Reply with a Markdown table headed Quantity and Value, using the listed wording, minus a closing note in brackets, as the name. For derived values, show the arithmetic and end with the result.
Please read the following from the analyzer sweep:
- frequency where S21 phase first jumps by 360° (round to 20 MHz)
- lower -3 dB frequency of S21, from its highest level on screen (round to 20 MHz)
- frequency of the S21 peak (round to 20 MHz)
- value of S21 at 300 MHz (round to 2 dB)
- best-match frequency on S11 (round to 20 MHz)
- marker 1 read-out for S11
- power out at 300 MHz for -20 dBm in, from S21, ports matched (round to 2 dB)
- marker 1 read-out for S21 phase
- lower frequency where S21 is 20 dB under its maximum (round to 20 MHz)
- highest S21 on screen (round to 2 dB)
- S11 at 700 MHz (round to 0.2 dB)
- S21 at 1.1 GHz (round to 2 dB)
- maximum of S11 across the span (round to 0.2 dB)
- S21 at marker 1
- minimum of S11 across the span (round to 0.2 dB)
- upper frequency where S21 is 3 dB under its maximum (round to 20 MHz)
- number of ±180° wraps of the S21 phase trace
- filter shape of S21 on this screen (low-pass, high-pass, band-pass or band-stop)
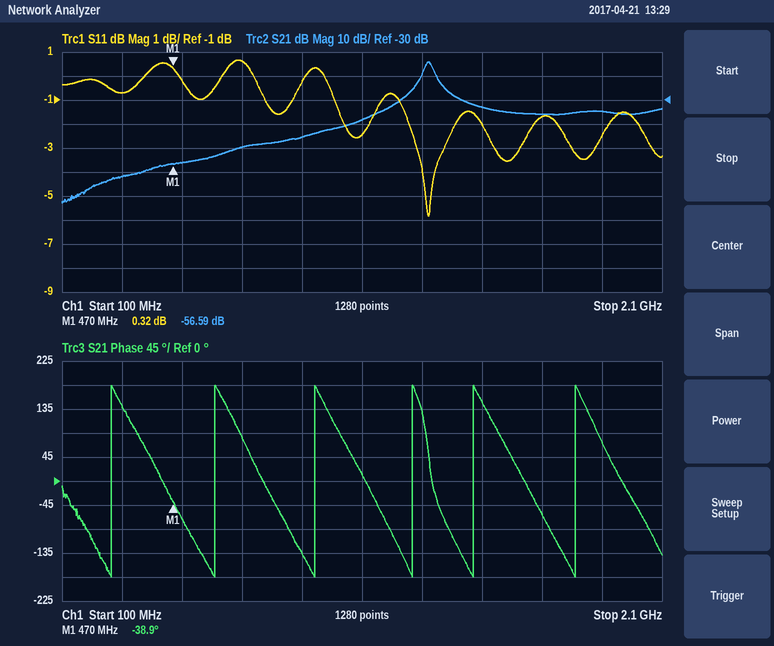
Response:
| Quantity | Value |
|---|---|
| frequency where S21 phase first jumps by 360° | 260 MHz |
| lower -3 dB frequency of S21, from its highest level on screen | 1.30 GHz |
| frequency of the S21 peak | 1.32 GHz |
| value of S21 at 300 MHz | -62 dB |
| best-match frequency on S11 | 1.32 GHz |
| marker 1 read-out for S11 | 0.32 dB |
| power out at 300 MHz for -20 dBm in, from S21, ports matched | -20 dBm + (-62 dB) = -82 dBm |
| marker 1 read-out for S21 phase | -38.9° |
| lower frequency where S21 is 20 dB under its maximum | 1.18 GHz |
| highest S21 on screen | -14 dB |
| S11 at 700 MHz | 0.6 dB |
| S21 at 1.1 GHz | -38 dB |
| maximum of S11 across the span | 0.6 dB |
| S21 at marker 1 | -56.59 dB |
| minimum of S11 across the span | -5.8 dB |
| upper frequency where S21 is 3 dB under its maximum | 1.34 GHz |
| number of ±180° wraps of the S21 phase trace | 6 |
| filter shape of S21 on this screen | band-pass |
